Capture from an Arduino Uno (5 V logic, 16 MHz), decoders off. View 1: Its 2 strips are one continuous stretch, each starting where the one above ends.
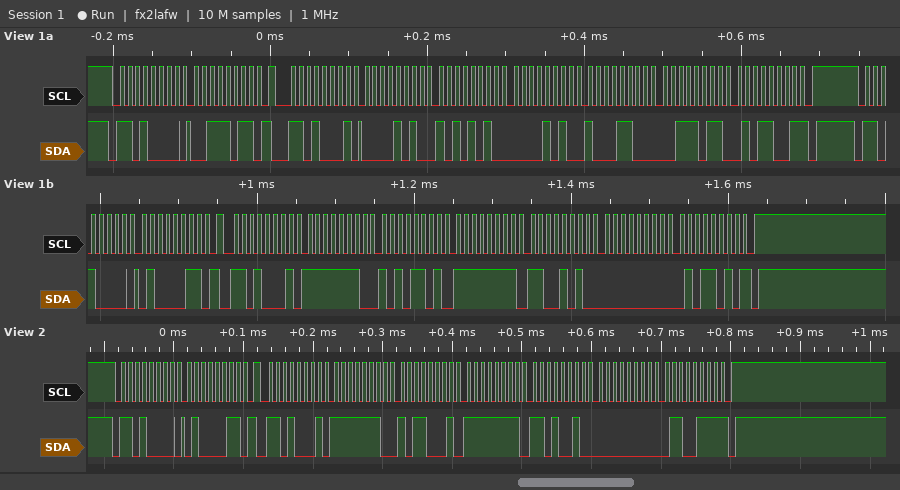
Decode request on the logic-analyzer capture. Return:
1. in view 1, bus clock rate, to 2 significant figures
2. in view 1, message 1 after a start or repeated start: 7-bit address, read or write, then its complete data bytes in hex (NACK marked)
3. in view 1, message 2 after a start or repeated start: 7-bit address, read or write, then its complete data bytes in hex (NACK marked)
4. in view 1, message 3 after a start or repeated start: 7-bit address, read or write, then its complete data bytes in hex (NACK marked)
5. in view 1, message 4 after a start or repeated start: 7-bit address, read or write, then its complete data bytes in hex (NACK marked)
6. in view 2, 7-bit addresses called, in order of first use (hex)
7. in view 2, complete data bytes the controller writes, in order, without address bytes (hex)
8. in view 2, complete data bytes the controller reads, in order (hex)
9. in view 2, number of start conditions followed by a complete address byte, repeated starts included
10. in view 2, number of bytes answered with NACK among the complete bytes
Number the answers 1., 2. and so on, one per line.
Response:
1. 100 kHz
2. 0x68 write: 3B
3. 0x68 read: 0A AA 0A 8C 3B 59 NACK
4. 0x68 write: 43
5. 0x68 read: FE AD FF CA 00 5A NACK
6. 0x68
7. 43
8. FE B1 FF D2 00 67
9. 2
10. 1
